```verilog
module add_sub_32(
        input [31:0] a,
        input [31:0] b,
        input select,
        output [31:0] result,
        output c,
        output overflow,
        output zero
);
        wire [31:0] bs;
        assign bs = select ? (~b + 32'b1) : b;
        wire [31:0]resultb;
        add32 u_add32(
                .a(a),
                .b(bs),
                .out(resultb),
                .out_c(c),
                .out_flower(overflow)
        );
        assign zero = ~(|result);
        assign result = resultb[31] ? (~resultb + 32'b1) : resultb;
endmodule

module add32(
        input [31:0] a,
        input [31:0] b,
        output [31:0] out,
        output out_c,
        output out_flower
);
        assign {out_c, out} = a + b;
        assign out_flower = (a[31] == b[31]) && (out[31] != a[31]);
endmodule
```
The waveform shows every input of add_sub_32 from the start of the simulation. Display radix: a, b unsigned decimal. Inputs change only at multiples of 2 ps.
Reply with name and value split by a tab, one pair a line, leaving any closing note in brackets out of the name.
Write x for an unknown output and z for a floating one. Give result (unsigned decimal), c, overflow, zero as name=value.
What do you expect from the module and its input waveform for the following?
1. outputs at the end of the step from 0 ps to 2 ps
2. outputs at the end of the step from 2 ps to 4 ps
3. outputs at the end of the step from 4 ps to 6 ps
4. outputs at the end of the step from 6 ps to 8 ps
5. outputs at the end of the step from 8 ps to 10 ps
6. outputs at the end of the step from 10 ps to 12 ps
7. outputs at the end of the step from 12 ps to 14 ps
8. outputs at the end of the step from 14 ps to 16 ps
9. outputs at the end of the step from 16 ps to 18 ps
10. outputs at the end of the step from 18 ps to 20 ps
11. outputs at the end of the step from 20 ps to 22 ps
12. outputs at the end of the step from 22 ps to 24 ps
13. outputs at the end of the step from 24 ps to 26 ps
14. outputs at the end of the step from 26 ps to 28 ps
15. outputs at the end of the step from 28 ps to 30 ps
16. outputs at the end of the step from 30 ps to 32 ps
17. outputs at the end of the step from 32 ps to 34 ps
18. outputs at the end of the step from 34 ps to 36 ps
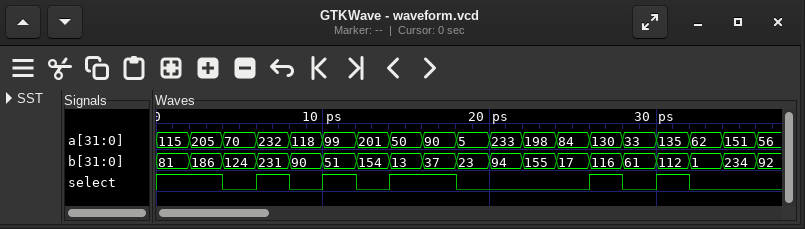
outputs at the end of the step from 0 ps to 2 ps	result=34, c=1, overflow=0, zero=0
outputs at the end of the step from 2 ps to 4 ps	result=19, c=1, overflow=0, zero=0
outputs at the end of the step from 4 ps to 6 ps	result=194, c=0, overflow=0, zero=0
outputs at the end of the step from 6 ps to 8 ps	result=1, c=1, overflow=0, zero=0
outputs at the end of the step from 8 ps to 10 ps	result=208, c=0, overflow=0, zero=0
outputs at the end of the step from 10 ps to 12 ps	result=48, c=1, overflow=0, zero=0
outputs at the end of the step from 12 ps to 14 ps	result=355, c=0, overflow=0, zero=0
outputs at the end of the step from 14 ps to 16 ps	result=37, c=1, overflow=0, zero=0
outputs at the end of the step from 16 ps to 18 ps	result=53, c=1, overflow=0, zero=0
outputs at the end of the step from 18 ps to 20 ps	result=28, c=0, overflow=0, zero=0
outputs at the end of the step from 20 ps to 22 ps	result=327, c=0, overflow=0, zero=0
outputs at the end of the step from 22 ps to 24 ps	result=353, c=0, overflow=0, zero=0
outputs at the end of the step from 24 ps to 26 ps	result=101, c=0, overflow=0, zero=0
outputs at the end of the step from 26 ps to 28 ps	result=14, c=1, overflow=0, zero=0
outputs at the end of the step from 28 ps to 30 ps	result=94, c=0, overflow=0, zero=0
outputs at the end of the step from 30 ps to 32 ps	result=23, c=1, overflow=0, zero=0
outputs at the end of the step from 32 ps to 34 ps	result=63, c=0, overflow=0, zero=0
outputs at the end of the step from 34 ps to 36 ps	result=385, c=0, overflow=0, zero=0
